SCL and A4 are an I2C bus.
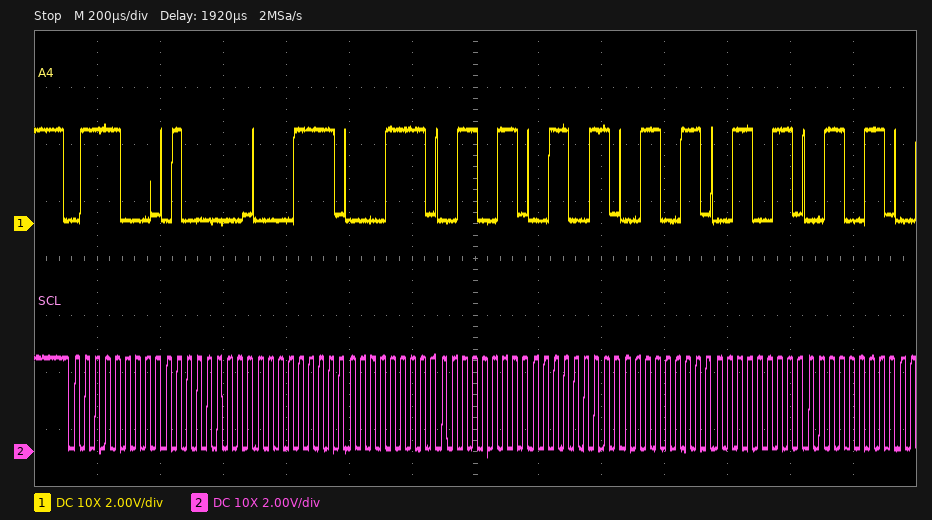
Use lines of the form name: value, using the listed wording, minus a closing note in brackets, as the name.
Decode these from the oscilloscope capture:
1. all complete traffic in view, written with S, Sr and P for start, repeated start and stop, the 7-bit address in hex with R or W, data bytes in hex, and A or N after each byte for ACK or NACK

all complete traffic in view, written with S, Sr and P for start, repeated start and stop, the 7-bit address in hex with R or W, data bytes in hex, and A or N after each byte for ACK or NACK: S 3CW A 40 A 0F A 0F A 33 A 33 A 33 A 33 A 33 A
